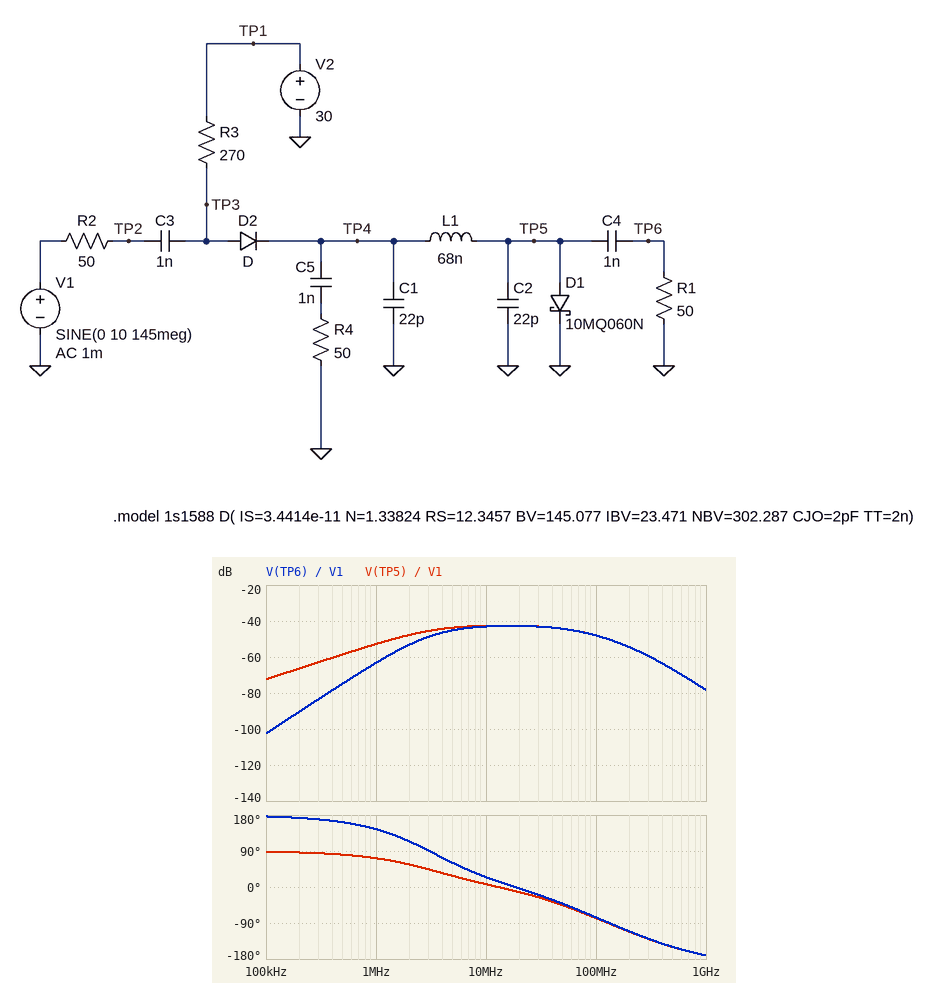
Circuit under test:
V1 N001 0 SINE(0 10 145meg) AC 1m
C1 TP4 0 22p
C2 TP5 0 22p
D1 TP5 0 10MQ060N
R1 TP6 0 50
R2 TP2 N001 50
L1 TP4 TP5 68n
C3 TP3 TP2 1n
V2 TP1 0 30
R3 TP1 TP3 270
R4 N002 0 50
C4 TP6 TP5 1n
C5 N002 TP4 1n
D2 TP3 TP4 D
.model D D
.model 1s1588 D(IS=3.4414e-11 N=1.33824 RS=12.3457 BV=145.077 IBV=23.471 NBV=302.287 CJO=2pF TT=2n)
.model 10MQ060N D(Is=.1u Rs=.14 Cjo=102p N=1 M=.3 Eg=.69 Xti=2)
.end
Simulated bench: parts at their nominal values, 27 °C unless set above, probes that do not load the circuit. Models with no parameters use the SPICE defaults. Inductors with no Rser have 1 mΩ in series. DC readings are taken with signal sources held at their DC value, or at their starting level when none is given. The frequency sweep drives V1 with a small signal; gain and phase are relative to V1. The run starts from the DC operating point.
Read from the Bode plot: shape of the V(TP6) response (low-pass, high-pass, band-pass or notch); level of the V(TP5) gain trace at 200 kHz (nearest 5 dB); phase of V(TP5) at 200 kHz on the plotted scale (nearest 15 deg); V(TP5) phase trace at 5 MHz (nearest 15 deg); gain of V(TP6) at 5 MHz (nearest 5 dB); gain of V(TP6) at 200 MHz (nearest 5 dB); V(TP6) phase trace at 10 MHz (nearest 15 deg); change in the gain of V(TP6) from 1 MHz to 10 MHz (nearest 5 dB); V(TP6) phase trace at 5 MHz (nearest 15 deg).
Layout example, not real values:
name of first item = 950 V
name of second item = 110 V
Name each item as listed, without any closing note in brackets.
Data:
shape of the V(TP6) response = band-pass
level of the V(TP5) gain trace at 200 kHz = -65 dB
phase of V(TP5) at 200 kHz on the plotted scale = 90 deg
V(TP5) phase trace at 5 MHz = 30 deg
gain of V(TP6) at 5 MHz = -45 dB
gain of V(TP6) at 200 MHz = -55 dB
V(TP6) phase trace at 10 MHz = 30 deg
change in the gain of V(TP6) from 1 MHz to 10 MHz = 20 dB
V(TP6) phase trace at 5 MHz = 60 deg
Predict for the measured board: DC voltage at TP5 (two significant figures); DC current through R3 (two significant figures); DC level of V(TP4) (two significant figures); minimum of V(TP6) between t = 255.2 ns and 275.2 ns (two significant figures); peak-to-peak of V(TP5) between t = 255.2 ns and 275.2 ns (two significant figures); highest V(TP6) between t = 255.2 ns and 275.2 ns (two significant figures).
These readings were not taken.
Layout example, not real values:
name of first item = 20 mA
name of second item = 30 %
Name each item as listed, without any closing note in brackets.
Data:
DC voltage at TP5 = 370 mV
DC current through R3 = 110 mA
DC level of V(TP4) = 370 mV
minimum of V(TP6) between t = 255.2 ns and 275.2 ns = -35 mV
peak-to-peak of V(TP5) between t = 255.2 ns and 275.2 ns = 63 mV
highest V(TP6) between t = 255.2 ns and 275.2 ns = 27 mV
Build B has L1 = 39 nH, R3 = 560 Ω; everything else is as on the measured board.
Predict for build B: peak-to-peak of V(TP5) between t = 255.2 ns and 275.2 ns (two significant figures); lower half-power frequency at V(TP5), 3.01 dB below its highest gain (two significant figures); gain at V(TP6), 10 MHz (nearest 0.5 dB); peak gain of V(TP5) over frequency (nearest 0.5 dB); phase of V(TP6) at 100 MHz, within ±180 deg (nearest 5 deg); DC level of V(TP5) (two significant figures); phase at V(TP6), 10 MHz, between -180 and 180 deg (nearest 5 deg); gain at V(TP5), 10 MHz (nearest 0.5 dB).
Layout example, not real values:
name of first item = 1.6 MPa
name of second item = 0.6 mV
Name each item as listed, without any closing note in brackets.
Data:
peak-to-peak of V(TP5) between t = 255.2 ns and 275.2 ns = 480 mV
lower half-power frequency at V(TP5), 3.01 dB below its highest gain = 3.0 MHz
gain at V(TP6), 10 MHz = -39.0 dB
peak gain of V(TP5) over frequency = -38.0 dB
phase of V(TP6) at 100 MHz, within ±180 deg = -55 deg
DC level of V(TP5) = 350 mV
phase at V(TP6), 10 MHz, between -180 and 180 deg = 30 deg
gain at V(TP5), 10 MHz = -38.5 dB
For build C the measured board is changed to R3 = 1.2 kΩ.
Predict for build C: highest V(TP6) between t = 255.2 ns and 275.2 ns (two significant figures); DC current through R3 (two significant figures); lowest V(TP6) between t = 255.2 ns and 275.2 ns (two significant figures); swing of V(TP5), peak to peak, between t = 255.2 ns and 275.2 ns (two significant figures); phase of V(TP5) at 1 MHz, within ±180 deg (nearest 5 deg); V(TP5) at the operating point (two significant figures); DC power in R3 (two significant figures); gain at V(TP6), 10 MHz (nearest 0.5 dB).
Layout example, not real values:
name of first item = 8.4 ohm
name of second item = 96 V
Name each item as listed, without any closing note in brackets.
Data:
highest V(TP6) between t = 255.2 ns and 275.2 ns = 47 mV
DC current through R3 = 24 mA
lowest V(TP6) between t = 255.2 ns and 275.2 ns = -84 mV
swing of V(TP5), peak to peak, between t = 255.2 ns and 275.2 ns = 130 mV
phase of V(TP5) at 1 MHz, within ±180 deg = 70 deg
V(TP5) at the operating point = 320 mV
DC power in R3 = 700 mW
gain at V(TP6), 10 MHz = -33.5 dB
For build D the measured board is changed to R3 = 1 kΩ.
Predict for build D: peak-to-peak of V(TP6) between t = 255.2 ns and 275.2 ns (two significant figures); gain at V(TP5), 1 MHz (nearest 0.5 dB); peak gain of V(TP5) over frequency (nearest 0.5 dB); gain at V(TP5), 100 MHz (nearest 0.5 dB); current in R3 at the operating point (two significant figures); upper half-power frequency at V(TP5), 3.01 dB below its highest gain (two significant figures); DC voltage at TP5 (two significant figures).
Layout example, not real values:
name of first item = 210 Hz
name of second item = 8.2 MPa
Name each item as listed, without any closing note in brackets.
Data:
peak-to-peak of V(TP6) between t = 255.2 ns and 275.2 ns = 130 mV
gain at V(TP5), 1 MHz = -44.0 dB
peak gain of V(TP5) over frequency = -34.5 dB
gain at V(TP5), 100 MHz = -39.0 dB
current in R3 at the operating point = 29 mA
upper half-power frequency at V(TP5), 3.01 dB below its highest gain = 74 MHz
DC voltage at TP5 = 330 mV
